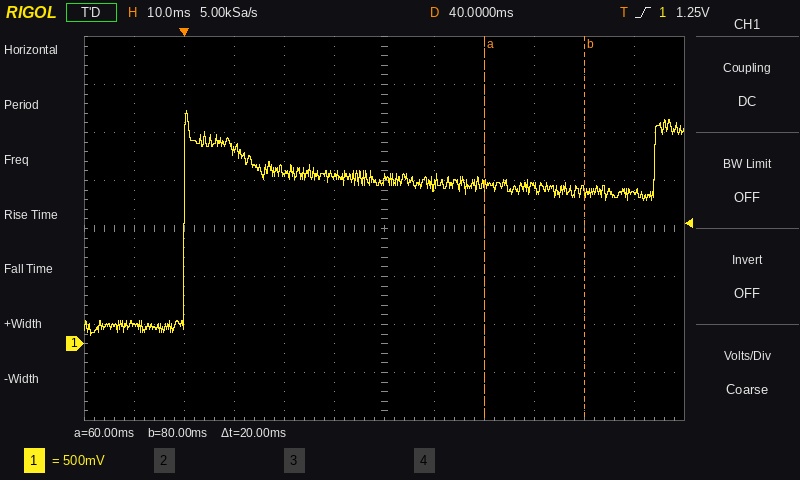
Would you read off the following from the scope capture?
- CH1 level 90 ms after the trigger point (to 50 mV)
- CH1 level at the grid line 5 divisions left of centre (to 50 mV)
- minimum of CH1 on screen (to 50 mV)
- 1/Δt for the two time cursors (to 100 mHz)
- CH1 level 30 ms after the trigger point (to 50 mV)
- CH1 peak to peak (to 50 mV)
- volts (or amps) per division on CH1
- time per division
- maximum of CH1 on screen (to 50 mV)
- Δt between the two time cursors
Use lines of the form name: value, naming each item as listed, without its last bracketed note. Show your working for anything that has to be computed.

CH1 level 90 ms after the trigger point: 1.60 V
CH1 level at the grid line 5 divisions left of centre: 200 mV
minimum of CH1 on screen: 100 mV
1/Δt for the two time cursors: 1 / 20 ms ≈ 50.0 Hz
CH1 level 30 ms after the trigger point: 1.75 V
CH1 peak to peak: 2.45 V − (100 mV) = 2.35 V
volts (or amps) per division on CH1: 500 mV
time per division: 10 ms
maximum of CH1 on screen: 2.45 V
Δt between the two time cursors: 20 ms
